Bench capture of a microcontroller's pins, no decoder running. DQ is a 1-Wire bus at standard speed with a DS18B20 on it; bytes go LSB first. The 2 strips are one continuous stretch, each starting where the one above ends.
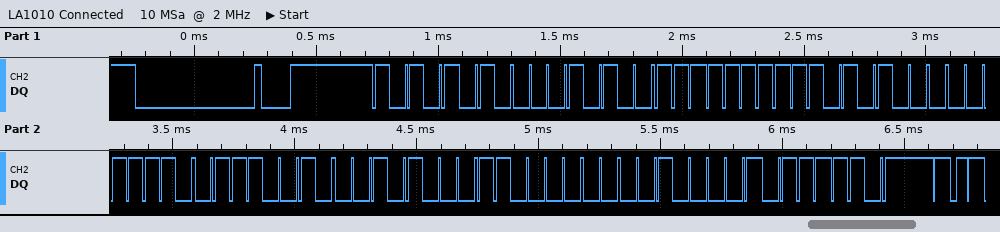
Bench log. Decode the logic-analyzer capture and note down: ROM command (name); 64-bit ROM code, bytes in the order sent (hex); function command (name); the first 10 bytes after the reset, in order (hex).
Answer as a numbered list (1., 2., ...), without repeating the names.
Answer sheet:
1. Match ROM
2. 28 FF 2B 78 4E 14 03 84
3. Read Scratchpad
4. 55 28 FF 2B 78 4E 14 03 84 BE
